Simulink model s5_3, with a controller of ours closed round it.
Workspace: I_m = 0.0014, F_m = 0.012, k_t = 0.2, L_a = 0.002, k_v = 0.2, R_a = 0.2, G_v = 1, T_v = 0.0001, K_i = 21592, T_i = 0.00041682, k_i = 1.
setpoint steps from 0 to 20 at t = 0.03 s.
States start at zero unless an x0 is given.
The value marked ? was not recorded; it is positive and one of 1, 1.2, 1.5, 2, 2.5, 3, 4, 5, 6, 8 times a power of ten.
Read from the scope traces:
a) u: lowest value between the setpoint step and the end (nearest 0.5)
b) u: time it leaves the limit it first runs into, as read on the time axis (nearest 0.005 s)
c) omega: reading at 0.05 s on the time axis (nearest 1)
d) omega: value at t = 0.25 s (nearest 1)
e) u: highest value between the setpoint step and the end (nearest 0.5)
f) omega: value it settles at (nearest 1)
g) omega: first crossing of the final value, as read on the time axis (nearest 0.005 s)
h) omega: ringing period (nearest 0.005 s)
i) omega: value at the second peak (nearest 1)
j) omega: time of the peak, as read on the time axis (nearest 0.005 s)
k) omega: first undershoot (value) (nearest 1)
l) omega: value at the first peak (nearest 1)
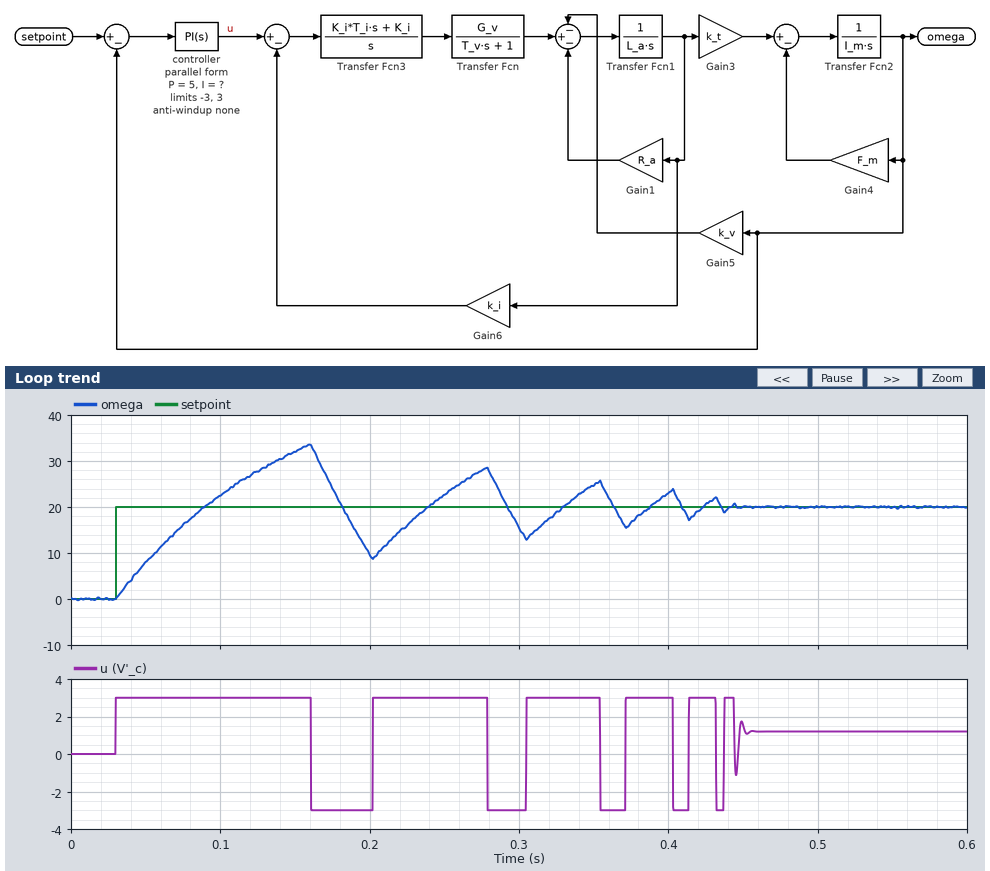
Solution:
-3.0
0.160 s
8
23
3.0
20
0.090 s
0.120 s
29
0.160 s
9
34
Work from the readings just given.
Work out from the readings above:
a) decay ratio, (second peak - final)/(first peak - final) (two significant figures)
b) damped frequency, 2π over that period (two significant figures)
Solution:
0.64
52 rad/s
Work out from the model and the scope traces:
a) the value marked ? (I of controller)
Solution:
6000
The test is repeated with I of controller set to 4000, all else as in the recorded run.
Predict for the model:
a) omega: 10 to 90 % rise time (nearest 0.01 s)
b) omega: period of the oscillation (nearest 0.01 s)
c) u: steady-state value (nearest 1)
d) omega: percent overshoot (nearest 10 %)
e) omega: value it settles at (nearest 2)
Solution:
0.05 s
0.11 s
1
70 %
20
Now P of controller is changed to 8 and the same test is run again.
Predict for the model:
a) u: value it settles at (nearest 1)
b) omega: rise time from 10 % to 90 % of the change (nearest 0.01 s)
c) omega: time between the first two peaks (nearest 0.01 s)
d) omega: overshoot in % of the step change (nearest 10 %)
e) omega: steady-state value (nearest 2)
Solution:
1
0.05 s
0.11 s
70 %
20
